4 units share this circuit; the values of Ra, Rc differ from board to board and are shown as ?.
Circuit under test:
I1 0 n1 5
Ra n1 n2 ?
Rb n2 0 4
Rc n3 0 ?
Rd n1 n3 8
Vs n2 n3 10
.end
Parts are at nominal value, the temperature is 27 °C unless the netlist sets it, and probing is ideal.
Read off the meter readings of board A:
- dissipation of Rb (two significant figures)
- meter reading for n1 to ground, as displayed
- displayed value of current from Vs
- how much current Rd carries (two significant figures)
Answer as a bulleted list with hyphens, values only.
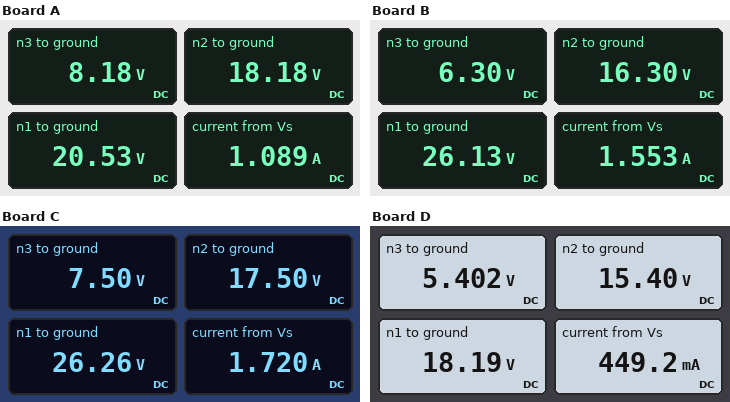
- 83 W
- 20.53 V
- 1.089 A
- 1.5 A
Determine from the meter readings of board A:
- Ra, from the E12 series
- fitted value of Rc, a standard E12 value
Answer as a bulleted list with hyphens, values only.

- 0.68 Ω
- 18 Ω
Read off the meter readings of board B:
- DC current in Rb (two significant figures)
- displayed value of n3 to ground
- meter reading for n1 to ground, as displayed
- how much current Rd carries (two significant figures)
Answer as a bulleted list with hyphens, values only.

- 4.1 A
- 6.30 V
- 26.13 V
- 2.5 A
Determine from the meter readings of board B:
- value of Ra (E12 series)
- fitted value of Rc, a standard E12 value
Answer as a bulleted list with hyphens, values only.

- 3.9 Ω
- 6.8 Ω
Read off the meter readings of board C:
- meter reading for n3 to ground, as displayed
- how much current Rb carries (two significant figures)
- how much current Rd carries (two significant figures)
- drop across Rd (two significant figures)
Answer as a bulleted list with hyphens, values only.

- 7.50 V
- 4.4 A
- 2.3 A
- 19 V
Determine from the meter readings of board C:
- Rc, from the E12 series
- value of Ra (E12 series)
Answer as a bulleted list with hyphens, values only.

- 12 Ω
- 3.3 Ω
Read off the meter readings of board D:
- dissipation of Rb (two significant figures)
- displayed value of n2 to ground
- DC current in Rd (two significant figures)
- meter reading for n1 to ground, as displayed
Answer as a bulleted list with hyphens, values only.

- 59 W
- 15.40 V
- 1.6 A
- 18.19 V
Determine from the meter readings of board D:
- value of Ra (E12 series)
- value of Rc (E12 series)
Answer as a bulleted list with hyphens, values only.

- 0.82 Ω
- 4.7 Ω
